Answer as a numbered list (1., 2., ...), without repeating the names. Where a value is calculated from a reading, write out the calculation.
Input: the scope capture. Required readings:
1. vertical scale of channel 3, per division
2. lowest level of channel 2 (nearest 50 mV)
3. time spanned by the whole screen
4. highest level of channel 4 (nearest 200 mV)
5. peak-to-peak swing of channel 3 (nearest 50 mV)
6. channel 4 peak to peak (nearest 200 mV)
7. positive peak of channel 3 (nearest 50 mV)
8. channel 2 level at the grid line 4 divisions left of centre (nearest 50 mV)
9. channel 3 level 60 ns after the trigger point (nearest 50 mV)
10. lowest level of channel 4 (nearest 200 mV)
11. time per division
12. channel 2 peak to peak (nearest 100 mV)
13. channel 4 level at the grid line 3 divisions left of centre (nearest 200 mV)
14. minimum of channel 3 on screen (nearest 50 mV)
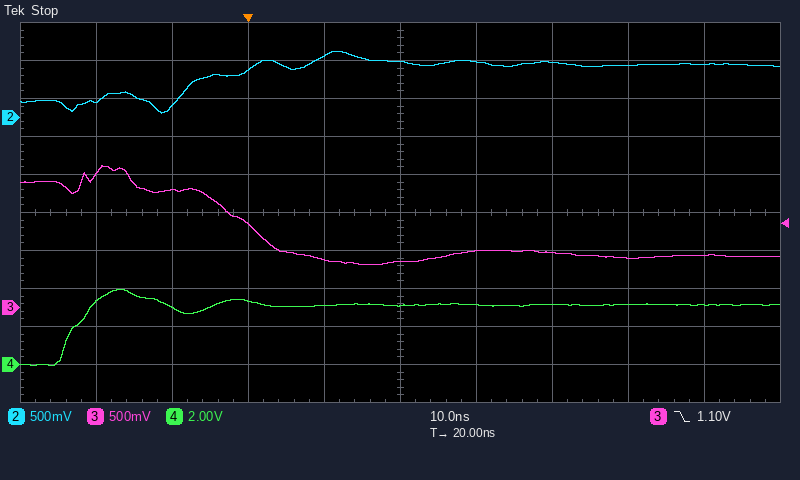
1. 500 mV
2. 50 mV
3. 100 ns
4. 4.0 V
5. 1.85 V − (550 mV) = 1.30 V
6. 4.0 V − (0.0 V) = 4.0 V
7. 1.85 V
8. 200 mV
9. 700 mV
10. 0.0 V
11. 10 ns
12. 800 mV
13. 3.0 V
14. 550 mV
